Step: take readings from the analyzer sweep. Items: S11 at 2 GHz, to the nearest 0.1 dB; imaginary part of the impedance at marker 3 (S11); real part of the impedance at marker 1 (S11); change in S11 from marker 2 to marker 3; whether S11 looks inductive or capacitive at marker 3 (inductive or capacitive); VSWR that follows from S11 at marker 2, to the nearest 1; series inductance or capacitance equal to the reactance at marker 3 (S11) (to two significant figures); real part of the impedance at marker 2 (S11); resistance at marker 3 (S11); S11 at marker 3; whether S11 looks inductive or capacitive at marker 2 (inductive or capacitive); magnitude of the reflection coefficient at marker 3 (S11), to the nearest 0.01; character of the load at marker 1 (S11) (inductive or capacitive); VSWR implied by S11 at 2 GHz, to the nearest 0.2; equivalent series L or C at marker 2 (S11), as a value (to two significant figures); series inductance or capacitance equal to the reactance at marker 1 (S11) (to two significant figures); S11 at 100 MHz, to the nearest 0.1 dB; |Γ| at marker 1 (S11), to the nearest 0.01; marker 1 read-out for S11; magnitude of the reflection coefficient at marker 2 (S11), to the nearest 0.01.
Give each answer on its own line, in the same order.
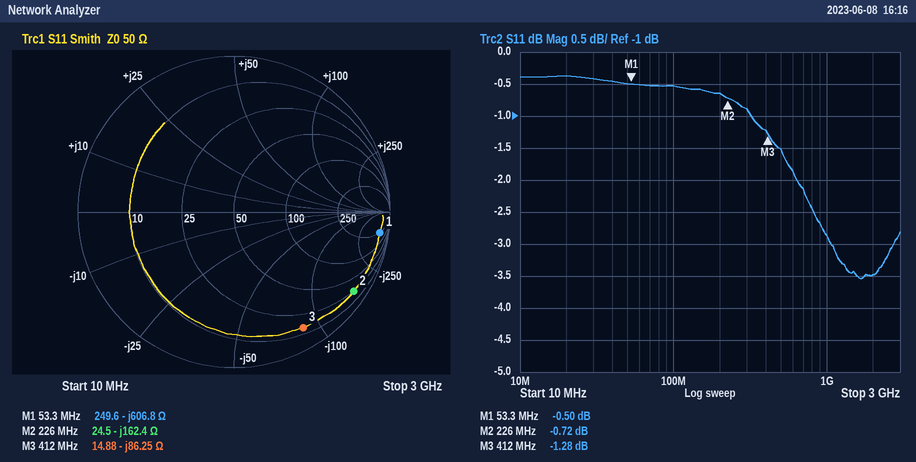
-3.5 dB
-86.25 Ω
249.6 Ω
-0.56 dB
capacitive
24
4.5 pF
24.5 Ω
14.88 Ω
-1.28 dB
capacitive
0.86
capacitive
5.0
4.3 pF
4.9 pF
-0.5 dB
0.94
-0.50 dB
0.92
